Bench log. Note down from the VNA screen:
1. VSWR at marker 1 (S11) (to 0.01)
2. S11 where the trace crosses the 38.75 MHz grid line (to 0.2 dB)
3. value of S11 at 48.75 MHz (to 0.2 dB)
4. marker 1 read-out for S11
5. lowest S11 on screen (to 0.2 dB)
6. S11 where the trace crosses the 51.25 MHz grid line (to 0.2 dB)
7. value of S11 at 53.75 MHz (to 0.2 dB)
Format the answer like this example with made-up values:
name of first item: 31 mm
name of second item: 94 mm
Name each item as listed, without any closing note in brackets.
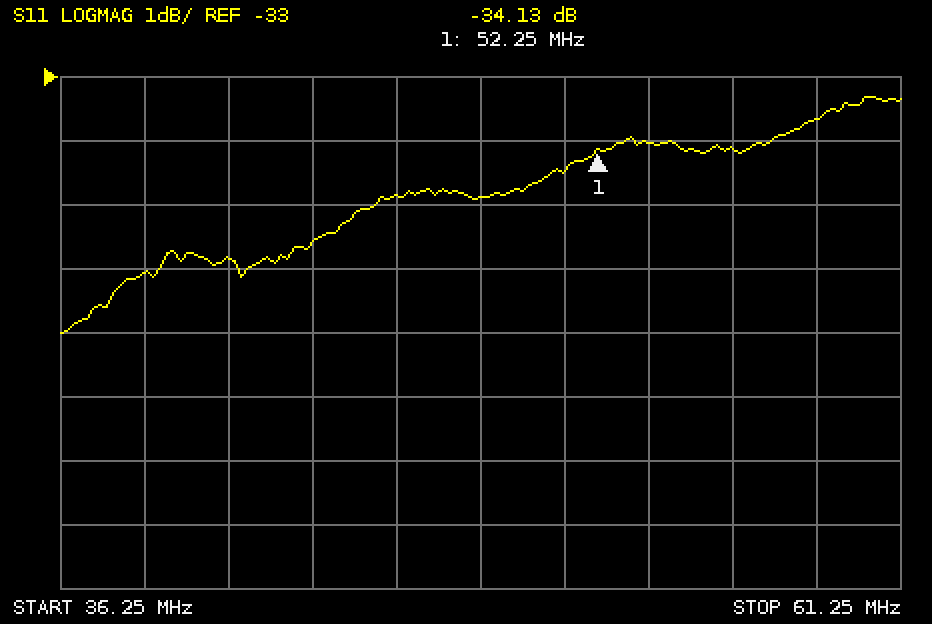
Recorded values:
VSWR at marker 1 (S11): 1.04
S11 where the trace crosses the 38.75 MHz grid line: -36.0 dB
value of S11 at 48.75 MHz: -34.8 dB
marker 1 read-out for S11: -34.13 dB
lowest S11 on screen: -37.0 dB
S11 where the trace crosses the 51.25 MHz grid line: -34.4 dB
value of S11 at 53.75 MHz: -34.0 dB
